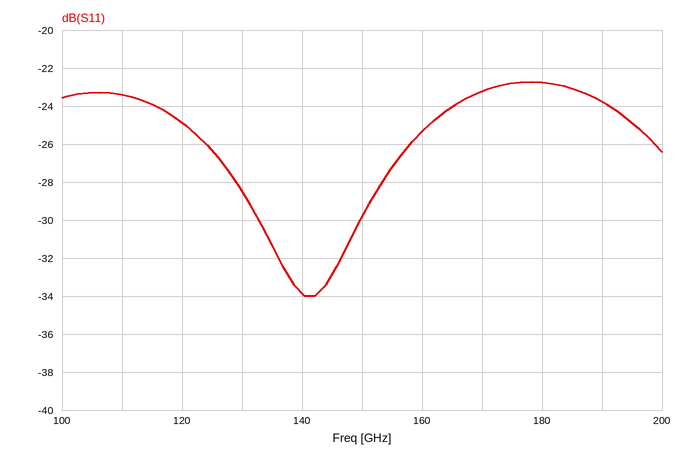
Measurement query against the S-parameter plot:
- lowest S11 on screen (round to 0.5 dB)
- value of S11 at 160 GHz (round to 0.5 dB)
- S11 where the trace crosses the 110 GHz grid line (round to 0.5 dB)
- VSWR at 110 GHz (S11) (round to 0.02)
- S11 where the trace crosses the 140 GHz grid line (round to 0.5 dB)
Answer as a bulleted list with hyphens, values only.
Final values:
- -34.0 dB
- -25.5 dB
- -23.5 dB
- 1.14
- -34.0 dB
